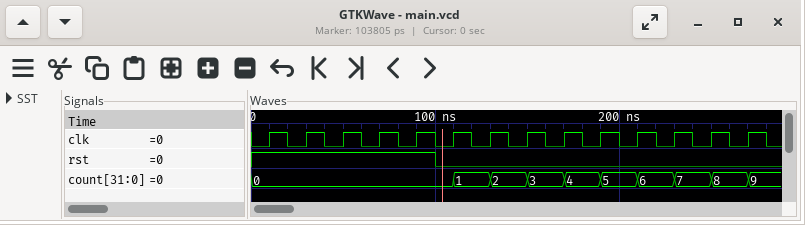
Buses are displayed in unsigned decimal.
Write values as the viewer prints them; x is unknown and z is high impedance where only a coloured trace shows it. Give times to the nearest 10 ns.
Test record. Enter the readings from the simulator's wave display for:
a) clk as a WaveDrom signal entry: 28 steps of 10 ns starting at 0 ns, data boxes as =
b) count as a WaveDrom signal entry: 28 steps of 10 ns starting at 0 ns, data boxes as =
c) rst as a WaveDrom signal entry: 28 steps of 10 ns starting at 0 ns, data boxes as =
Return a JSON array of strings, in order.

["{name: 'clk', wave: '0101010101010101010101010101'}", "{name: 'count', wave: '=..........=.=.=.=.=.=.=.=.=', data: '0 1 2 3 4 5 6 7 8 9'}", "{name: 'rst', wave: '1.........0.................'}"]
